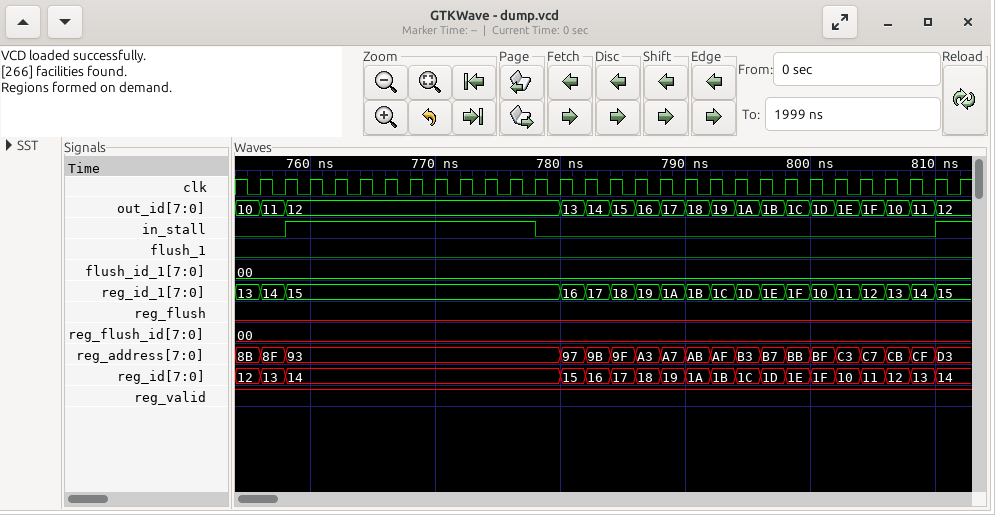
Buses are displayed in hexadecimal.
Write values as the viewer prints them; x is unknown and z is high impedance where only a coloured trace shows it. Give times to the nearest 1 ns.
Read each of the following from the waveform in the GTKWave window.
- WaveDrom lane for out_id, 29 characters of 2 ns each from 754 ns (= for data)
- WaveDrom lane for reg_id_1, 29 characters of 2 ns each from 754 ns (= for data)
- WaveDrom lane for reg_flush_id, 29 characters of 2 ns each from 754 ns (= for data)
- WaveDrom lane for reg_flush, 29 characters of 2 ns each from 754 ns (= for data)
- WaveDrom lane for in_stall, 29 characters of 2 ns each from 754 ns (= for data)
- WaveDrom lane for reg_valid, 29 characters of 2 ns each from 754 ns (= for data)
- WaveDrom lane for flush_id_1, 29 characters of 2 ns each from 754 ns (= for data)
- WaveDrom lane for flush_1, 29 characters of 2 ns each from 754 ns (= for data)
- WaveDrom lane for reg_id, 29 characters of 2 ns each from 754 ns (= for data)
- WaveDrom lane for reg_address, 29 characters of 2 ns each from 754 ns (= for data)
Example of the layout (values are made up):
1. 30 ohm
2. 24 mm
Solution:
1. {name: 'out_id', wave: '===..........================', data: '10 11 12 13 14 15 16 17 18 19 1A 1B 1C 1D 1E 1F 10 11 12'}
2. {name: 'reg_id_1', wave: '===..........================', data: '13 14 15 16 17 18 19 1A 1B 1C 1D 1E 1F 10 11 12 13 14 15'}
3. {name: 'reg_flush_id', wave: '=............................', data: '00'}
4. {name: 'reg_flush', wave: '0............................'}
5. {name: 'in_stall', wave: '0.1.........0...............1'}
6. {name: 'reg_valid', wave: '1............................'}
7. {name: 'flush_id_1', wave: '=............................', data: '00'}
8. {name: 'flush_1', wave: '0............................'}
9. {name: 'reg_id', wave: '===..........================', data: '12 13 14 15 16 17 18 19 1A 1B 1C 1D 1E 1F 10 11 12 13 14'}
10. {name: 'reg_address', wave: '===..........================', data: '8B 8F 93 97 9B 9F A3 A7 AB AF B3 B7 BB BF C3 C7 CB CF D3'}
